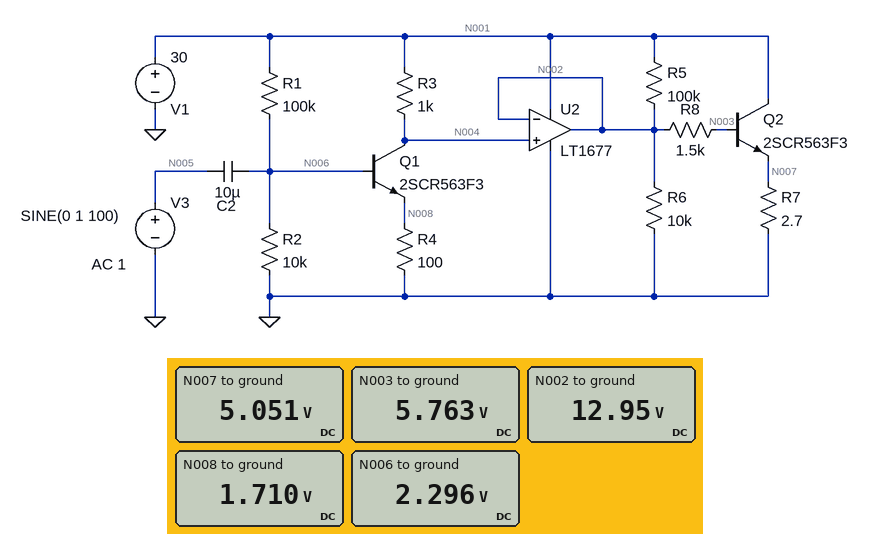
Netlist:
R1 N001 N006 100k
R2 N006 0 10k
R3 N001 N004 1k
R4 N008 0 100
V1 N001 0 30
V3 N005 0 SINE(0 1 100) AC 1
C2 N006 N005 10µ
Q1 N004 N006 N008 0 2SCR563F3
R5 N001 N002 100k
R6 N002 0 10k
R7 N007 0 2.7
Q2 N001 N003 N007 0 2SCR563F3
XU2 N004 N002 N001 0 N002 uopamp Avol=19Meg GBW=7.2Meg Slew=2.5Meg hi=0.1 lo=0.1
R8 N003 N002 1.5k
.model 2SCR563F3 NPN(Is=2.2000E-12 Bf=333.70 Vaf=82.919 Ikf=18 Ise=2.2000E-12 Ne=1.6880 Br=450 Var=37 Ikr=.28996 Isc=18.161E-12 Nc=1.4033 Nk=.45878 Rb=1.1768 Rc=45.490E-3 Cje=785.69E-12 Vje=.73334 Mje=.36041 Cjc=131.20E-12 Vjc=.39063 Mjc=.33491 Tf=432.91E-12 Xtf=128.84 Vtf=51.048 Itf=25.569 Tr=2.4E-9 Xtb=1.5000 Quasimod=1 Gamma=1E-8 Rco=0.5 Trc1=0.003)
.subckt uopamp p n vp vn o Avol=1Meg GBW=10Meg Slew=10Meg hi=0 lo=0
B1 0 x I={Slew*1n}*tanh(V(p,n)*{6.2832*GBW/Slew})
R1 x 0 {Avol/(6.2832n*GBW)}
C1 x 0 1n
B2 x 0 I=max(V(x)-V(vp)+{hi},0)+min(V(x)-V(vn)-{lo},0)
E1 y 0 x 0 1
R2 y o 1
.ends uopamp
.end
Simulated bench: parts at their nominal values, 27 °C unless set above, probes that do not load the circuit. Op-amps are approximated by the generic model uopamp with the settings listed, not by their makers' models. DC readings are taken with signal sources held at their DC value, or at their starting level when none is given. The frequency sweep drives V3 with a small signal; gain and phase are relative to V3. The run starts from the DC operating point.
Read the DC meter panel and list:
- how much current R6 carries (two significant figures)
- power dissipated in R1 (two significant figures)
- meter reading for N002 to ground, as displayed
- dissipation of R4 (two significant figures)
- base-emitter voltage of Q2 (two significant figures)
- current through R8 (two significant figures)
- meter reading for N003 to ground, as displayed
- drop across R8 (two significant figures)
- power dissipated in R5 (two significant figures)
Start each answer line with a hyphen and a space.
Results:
- 1.3 mA
- 7.7 mW
- 12.95 V
- 29 mW
- 710 mV
- 4.8 mA
- 5.763 V
- 7.2 V
- 2.9 mW
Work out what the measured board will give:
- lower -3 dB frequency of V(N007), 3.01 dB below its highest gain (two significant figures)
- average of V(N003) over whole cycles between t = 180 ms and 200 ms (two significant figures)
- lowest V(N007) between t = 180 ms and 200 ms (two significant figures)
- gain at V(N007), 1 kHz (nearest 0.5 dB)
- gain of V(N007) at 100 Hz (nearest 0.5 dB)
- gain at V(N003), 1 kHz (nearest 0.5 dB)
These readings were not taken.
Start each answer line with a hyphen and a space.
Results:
- 2.3 Hz
- 5.7 V
- 1.1 V
- 11.5 dB
- 11.5 dB
- 11.5 dB
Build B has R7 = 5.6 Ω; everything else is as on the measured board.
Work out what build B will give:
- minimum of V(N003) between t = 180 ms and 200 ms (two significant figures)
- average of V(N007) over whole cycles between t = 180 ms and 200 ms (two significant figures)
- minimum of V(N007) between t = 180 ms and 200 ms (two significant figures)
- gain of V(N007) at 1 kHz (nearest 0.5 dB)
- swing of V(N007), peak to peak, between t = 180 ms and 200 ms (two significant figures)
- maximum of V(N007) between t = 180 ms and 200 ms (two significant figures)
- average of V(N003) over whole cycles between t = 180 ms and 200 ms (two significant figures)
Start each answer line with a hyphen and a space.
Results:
- 2.3 V
- 7.2 V
- 1.6 V
- 15.0 dB
- 11 V
- 13 V
- 7.9 V
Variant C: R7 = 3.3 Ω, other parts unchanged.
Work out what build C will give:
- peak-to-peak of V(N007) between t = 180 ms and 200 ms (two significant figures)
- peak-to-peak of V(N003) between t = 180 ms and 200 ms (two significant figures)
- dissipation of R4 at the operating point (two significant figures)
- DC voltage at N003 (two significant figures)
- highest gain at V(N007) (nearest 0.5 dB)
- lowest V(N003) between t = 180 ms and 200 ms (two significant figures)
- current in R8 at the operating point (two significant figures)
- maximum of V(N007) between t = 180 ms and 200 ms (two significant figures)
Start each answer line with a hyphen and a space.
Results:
- 8.4 V
- 8.5 V
- 29 mW
- 6.4 V
- 12.5 dB
- 1.9 V
- 4.4 mA
- 9.7 V
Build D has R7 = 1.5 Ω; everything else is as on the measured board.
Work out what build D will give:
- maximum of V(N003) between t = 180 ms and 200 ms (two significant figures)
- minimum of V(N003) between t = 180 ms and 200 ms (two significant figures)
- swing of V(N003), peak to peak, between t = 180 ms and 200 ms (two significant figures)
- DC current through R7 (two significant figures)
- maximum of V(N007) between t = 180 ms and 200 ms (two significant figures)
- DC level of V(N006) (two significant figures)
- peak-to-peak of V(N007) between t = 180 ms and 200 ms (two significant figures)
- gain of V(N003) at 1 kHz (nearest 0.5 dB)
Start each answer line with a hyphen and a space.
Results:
- 6.5 V
- 1.5 V
- 5.1 V
- 2.3 A
- 5.8 V
- 2.3 V
- 5.0 V
- 8.0 dB
